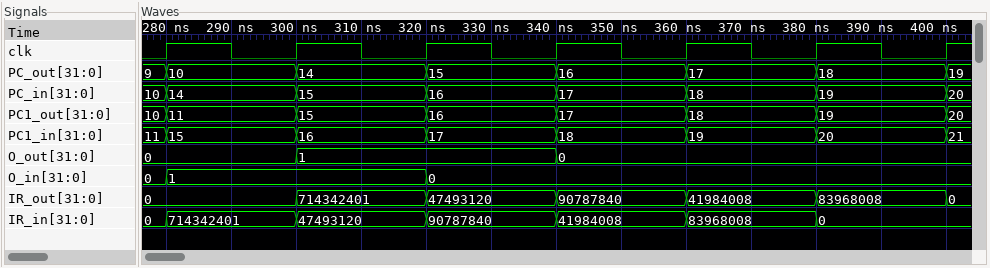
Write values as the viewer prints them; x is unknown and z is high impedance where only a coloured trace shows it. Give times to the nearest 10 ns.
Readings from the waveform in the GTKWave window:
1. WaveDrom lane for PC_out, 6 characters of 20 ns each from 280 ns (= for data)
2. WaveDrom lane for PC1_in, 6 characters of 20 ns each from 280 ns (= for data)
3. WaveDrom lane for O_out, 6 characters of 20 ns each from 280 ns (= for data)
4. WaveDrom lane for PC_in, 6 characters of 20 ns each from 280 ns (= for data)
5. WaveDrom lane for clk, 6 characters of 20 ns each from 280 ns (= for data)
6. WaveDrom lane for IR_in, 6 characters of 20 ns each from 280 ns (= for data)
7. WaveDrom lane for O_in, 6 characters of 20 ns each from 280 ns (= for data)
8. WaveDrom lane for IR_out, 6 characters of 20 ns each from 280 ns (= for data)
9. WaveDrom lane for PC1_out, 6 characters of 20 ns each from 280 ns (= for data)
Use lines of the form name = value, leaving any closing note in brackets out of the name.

WaveDrom lane for PC_out, 6 characters of 20 ns each from 280 ns = {name: 'PC_out', wave: '======', data: '10 14 15 16 17 18'}
WaveDrom lane for PC1_in, 6 characters of 20 ns each from 280 ns = {name: 'PC1_in', wave: '======', data: '15 16 17 18 19 20'}
WaveDrom lane for O_out, 6 characters of 20 ns each from 280 ns = {name: 'O_out', wave: '==.=..', data: '0 1 0'}
WaveDrom lane for PC_in, 6 characters of 20 ns each from 280 ns = {name: 'PC_in', wave: '======', data: '14 15 16 17 18 19'}
WaveDrom lane for clk, 6 characters of 20 ns each from 280 ns = {name: 'clk', wave: 'p.....'}
WaveDrom lane for IR_in, 6 characters of 20 ns each from 280 ns = {name: 'IR_in', wave: '======', data: '714342401 47493120 90787840 41984008 83968008 0'}
WaveDrom lane for O_in, 6 characters of 20 ns each from 280 ns = {name: 'O_in', wave: '=.=...', data: '1 0'}
WaveDrom lane for IR_out, 6 characters of 20 ns each from 280 ns = {name: 'IR_out', wave: '======', data: '0 714342401 47493120 90787840 41984008 83968008'}
WaveDrom lane for PC1_out, 6 characters of 20 ns each from 280 ns = {name: 'PC1_out', wave: '======', data: '11 15 16 17 18 19'}
